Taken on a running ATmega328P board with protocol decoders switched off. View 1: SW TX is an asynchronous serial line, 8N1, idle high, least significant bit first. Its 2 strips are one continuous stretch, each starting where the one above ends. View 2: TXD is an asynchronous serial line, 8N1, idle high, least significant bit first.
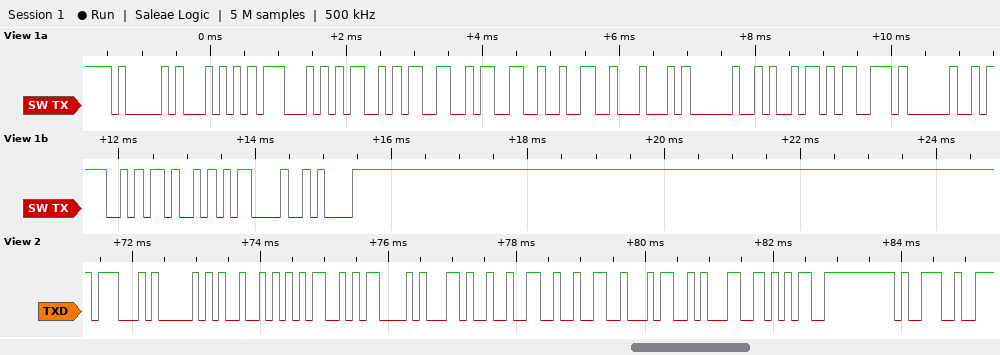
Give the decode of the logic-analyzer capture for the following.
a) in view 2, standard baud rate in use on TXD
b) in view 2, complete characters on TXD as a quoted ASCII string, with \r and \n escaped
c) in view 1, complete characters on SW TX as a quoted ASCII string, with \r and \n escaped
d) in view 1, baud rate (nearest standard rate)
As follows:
9600 baud
"GPRMC,224159"
"ATGM332D is OK\r\n"
9600 baud
